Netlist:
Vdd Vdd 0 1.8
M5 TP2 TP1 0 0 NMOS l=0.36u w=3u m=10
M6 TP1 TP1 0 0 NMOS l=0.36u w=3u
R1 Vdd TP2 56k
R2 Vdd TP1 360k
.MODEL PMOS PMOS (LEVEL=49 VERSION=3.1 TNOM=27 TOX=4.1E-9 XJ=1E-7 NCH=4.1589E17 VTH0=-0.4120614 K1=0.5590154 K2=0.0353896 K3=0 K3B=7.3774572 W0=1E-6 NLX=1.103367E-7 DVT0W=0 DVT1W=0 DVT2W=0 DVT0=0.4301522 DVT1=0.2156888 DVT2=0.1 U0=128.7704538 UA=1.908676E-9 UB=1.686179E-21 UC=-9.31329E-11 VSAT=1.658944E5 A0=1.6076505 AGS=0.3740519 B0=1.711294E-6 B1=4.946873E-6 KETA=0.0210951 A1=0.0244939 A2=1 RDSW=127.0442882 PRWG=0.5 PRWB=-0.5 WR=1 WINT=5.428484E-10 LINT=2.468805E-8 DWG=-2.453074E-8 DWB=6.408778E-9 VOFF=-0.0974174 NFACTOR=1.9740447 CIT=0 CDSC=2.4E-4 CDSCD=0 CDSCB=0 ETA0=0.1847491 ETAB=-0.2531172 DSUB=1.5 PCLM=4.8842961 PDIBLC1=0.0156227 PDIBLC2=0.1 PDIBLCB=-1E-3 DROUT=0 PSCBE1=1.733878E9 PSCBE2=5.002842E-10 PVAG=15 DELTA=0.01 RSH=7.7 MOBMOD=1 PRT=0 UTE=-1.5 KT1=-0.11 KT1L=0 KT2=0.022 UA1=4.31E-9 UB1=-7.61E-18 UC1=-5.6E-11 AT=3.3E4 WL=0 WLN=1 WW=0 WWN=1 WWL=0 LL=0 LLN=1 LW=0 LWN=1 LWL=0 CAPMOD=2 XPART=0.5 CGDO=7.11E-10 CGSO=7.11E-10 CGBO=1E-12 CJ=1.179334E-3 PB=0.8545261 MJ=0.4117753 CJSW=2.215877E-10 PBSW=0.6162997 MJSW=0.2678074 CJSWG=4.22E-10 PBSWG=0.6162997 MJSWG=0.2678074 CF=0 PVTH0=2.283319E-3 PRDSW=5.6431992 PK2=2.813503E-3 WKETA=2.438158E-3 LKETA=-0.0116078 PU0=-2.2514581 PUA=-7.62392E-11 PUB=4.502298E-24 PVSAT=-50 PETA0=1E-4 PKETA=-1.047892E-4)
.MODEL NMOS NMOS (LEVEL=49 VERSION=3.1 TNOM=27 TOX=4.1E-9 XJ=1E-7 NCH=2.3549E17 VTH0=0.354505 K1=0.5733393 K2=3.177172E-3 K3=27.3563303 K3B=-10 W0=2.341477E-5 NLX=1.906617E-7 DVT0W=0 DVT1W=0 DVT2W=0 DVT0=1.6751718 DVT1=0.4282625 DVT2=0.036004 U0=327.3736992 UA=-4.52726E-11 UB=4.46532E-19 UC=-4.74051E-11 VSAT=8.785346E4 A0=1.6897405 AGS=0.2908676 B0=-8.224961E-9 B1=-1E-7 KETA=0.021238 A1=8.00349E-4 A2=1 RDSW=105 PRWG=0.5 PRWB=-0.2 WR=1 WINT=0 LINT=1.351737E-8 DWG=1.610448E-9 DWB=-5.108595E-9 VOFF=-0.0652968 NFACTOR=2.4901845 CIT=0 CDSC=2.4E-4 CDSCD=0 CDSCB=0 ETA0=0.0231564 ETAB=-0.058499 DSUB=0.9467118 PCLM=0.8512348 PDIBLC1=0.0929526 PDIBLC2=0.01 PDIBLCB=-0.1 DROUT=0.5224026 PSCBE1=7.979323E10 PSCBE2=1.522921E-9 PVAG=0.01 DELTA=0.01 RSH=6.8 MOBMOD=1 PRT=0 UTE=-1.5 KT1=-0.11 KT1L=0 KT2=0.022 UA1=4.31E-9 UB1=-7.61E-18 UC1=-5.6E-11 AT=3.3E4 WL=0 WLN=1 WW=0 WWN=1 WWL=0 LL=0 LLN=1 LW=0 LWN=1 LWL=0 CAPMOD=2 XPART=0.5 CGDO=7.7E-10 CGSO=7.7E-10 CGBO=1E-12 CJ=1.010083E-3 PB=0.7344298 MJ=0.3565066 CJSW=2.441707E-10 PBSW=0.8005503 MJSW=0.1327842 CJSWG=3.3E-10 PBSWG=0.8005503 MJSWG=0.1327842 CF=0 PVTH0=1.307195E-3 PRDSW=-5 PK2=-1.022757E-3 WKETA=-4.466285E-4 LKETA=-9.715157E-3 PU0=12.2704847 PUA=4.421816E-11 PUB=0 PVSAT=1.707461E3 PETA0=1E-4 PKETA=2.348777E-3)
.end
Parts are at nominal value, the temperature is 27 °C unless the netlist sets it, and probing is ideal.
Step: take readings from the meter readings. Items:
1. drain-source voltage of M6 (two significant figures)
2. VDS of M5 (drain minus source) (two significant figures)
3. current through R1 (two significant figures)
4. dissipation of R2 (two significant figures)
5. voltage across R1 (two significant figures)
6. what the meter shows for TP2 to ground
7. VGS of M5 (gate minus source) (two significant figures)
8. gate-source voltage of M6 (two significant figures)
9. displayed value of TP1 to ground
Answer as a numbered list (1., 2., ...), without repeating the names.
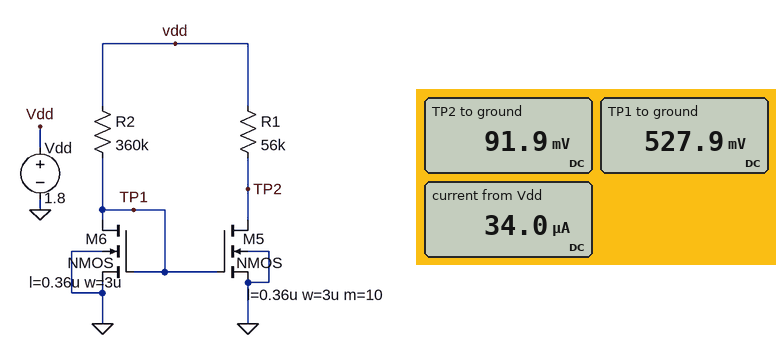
1. 530 mV
2. 92 mV
3. 31 µA
4. 4.5 µW
5. 1.7 V
6. 91.9 mV
7. 530 mV
8. 530 mV
9. 527.9 mV
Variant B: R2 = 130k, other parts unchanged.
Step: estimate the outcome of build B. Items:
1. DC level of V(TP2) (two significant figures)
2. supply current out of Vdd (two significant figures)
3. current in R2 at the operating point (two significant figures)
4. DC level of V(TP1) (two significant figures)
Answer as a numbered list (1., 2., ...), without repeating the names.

1. 22 mV
2. 41 µA
3. 9.4 µA
4. 580 mV
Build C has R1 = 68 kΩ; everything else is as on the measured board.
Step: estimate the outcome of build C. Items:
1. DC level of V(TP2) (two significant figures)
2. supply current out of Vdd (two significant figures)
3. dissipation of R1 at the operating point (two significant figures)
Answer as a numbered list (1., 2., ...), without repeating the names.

1. 51 mV
2. 29 µA
3. 45 µW
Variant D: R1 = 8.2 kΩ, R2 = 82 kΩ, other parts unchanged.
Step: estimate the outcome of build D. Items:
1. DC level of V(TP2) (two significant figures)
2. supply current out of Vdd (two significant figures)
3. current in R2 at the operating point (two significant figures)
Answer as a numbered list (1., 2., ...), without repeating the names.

1. 600 mV
2. 160 µA
3. 15 µA
